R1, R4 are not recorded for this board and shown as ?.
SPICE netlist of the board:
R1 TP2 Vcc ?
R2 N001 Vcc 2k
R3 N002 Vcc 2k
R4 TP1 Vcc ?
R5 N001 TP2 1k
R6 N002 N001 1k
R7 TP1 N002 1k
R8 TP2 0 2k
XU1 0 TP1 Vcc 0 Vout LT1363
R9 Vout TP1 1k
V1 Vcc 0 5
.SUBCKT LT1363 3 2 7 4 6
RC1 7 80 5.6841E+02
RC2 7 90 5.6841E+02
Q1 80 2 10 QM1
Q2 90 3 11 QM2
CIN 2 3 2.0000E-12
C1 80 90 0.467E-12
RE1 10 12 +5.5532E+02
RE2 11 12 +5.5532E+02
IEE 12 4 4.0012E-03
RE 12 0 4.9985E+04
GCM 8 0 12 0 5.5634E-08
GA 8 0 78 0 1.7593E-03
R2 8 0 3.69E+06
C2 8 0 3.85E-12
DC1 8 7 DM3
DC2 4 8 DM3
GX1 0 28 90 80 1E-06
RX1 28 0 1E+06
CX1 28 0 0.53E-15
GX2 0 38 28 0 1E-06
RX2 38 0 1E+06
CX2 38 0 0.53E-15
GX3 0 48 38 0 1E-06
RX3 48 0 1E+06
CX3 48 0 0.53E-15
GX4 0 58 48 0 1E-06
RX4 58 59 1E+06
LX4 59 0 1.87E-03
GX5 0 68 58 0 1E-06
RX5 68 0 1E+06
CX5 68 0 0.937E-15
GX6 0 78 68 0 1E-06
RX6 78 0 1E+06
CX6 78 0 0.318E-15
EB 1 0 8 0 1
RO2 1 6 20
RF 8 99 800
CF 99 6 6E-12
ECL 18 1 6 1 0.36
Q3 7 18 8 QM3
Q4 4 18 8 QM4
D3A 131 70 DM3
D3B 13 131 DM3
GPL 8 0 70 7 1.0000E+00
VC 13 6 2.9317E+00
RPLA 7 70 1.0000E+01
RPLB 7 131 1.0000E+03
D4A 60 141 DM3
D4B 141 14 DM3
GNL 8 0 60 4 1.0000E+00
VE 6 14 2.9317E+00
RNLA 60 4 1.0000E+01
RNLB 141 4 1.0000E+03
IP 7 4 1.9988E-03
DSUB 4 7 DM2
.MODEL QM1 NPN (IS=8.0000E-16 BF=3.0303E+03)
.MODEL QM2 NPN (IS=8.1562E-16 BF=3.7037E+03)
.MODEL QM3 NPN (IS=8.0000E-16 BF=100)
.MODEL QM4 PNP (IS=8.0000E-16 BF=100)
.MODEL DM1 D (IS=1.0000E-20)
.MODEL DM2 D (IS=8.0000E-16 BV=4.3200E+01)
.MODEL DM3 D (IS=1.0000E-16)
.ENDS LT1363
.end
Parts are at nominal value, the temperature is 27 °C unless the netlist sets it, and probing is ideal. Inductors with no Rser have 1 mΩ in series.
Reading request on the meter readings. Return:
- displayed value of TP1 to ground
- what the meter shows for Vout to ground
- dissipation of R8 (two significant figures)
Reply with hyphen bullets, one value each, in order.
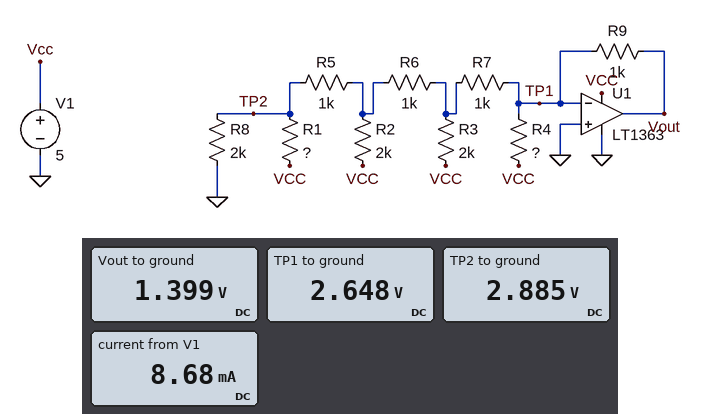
- 2.648 V
- 1.399 V
- 4.2 mW
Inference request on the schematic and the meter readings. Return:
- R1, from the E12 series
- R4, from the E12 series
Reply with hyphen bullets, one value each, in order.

- 2.7 kΩ
- 5.6 kΩ
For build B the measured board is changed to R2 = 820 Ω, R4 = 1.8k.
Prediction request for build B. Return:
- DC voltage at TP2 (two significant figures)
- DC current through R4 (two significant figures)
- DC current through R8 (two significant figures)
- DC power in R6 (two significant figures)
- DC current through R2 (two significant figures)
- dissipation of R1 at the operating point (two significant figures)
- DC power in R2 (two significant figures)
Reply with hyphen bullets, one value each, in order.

- 3.2 V
- 1.0 mA
- 1.6 mA
- 37 µW
- 1.1 mA
- 1.2 mW
- 1.0 mW
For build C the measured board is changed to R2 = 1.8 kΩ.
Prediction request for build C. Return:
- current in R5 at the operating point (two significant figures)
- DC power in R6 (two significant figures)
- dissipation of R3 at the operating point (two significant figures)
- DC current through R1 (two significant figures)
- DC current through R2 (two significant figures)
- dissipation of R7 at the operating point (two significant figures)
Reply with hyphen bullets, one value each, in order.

- 680 µA
- 9.0 µW
- 1.1 mW
- 770 µA
- 780 µA
- 710 µW
